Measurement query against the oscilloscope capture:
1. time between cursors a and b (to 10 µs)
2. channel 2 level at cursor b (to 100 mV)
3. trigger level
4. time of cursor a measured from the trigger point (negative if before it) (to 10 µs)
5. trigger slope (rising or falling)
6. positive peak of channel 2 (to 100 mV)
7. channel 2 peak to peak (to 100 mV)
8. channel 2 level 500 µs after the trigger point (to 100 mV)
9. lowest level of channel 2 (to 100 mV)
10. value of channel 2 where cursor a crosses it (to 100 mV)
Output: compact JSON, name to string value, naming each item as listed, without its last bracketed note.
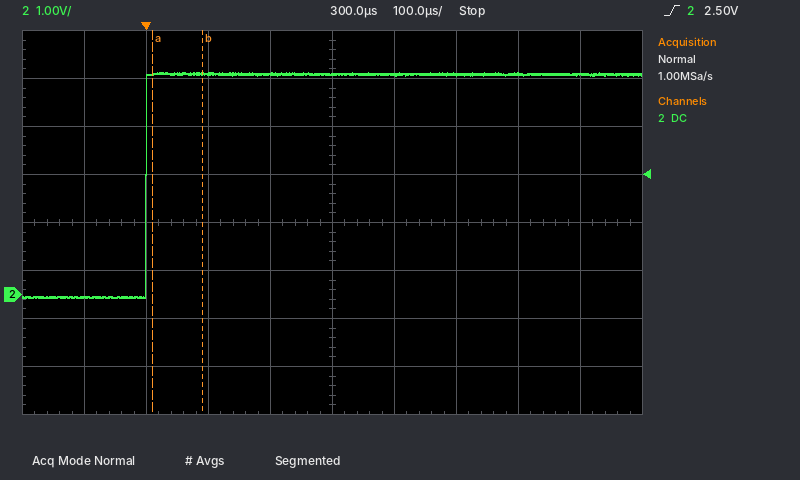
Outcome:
{"time between cursors a and b": "80 µs", "channel 2 level at cursor b": "4.6 V", "trigger level": "2.50 V", "time of cursor a measured from the trigger point (negative if before it)": "+10 µs", "trigger slope": "rising", "positive peak of channel 2": "4.6 V", "channel 2 peak to peak": "4.7 V", "channel 2 level 500 µs after the trigger point": "4.6 V", "lowest level of channel 2": "-100 mV", "value of channel 2 where cursor a crosses it": "4.6 V"}
